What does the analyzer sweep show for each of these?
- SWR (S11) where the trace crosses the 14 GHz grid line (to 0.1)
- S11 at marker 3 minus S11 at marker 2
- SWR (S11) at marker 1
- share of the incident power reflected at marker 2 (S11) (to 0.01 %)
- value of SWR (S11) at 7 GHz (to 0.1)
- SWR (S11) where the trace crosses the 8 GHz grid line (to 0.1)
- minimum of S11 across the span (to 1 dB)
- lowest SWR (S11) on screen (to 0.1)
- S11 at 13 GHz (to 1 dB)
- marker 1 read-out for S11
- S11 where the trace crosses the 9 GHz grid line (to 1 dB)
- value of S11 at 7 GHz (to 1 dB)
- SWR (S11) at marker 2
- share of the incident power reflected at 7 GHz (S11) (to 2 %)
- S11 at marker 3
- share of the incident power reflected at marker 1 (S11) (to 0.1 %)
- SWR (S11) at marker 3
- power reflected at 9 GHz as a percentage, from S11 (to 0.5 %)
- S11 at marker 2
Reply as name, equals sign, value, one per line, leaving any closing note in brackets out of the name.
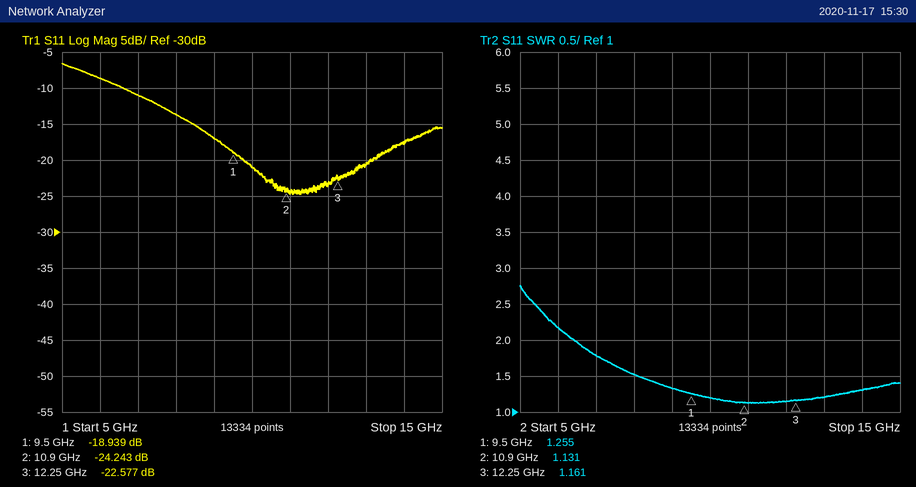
SWR (S11) where the trace crosses the 14 GHz grid line = 1.3
S11 at marker 3 minus S11 at marker 2 = 1.666 dB
SWR (S11) at marker 1 = 1.255
share of the incident power reflected at marker 2 (S11) = 0.38 %
value of SWR (S11) at 7 GHz = 1.8
SWR (S11) where the trace crosses the 8 GHz grid line = 1.5
minimum of S11 across the span = -25 dB
lowest SWR (S11) on screen = 1.1
S11 at 13 GHz = -21 dB
marker 1 read-out for S11 = -18.939 dB
S11 where the trace crosses the 9 GHz grid line = -17 dB
value of S11 at 7 GHz = -11 dB
SWR (S11) at marker 2 = 1.131
share of the incident power reflected at 7 GHz (S11) = 8 %
S11 at marker 3 = -22.577 dB
share of the incident power reflected at marker 1 (S11) = 1.3 %
SWR (S11) at marker 3 = 1.161
power reflected at 9 GHz as a percentage, from S11 = 2.0 %
S11 at marker 2 = -24.243 dB
